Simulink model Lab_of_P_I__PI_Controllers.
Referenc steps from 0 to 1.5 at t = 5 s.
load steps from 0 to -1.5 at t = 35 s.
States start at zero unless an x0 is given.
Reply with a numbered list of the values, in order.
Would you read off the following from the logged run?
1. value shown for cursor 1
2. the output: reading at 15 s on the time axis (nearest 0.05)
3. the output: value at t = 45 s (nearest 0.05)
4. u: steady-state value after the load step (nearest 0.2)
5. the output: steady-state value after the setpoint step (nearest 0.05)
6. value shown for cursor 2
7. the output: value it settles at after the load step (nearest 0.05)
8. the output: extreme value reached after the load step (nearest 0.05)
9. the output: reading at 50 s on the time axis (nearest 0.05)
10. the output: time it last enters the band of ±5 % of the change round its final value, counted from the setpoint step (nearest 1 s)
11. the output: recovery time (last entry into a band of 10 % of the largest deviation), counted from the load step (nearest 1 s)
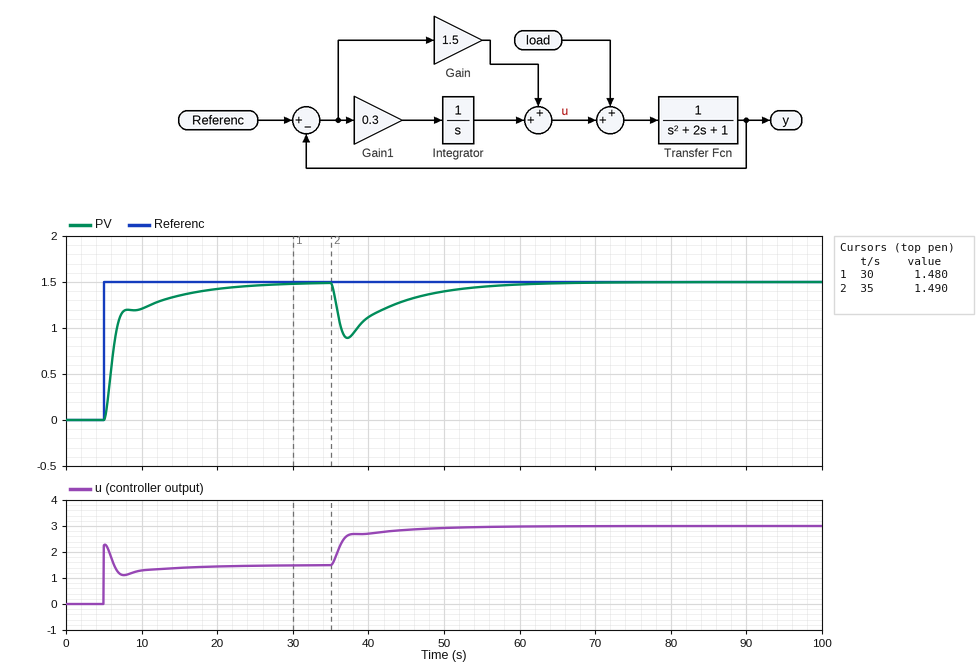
1. 1.480
2. 1.35
3. 1.30
4. 3.0
5. 1.50
6. 1.490
7. 1.50
8. 0.90
9. 1.40
10. 15 s
11. 19 s
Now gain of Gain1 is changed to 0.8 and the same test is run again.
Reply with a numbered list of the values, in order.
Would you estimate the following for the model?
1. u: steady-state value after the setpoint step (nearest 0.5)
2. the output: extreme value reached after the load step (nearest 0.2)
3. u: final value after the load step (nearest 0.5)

1. 1.5
2. 1.0
3. 3.0
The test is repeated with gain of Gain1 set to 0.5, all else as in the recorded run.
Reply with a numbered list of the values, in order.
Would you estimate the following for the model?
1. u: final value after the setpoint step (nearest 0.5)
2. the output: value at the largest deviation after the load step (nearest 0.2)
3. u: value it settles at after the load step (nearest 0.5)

1. 1.5
2. 1.0
3. 3.0
